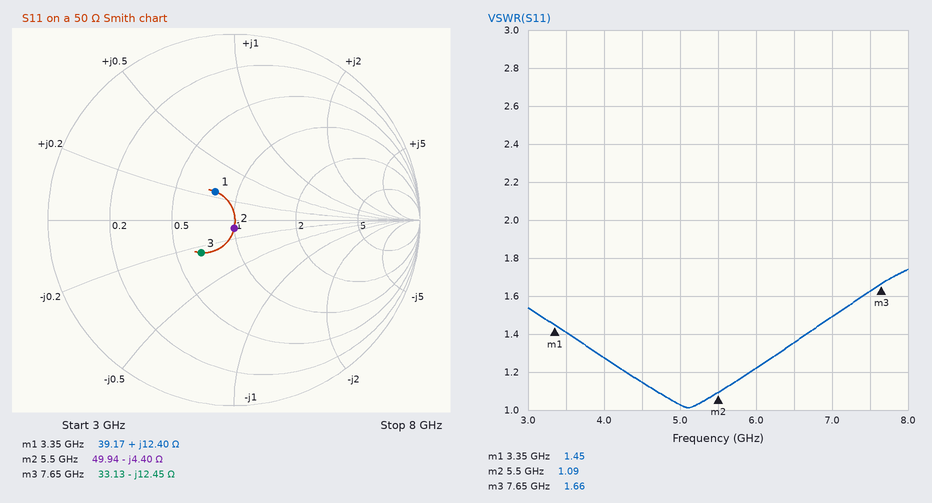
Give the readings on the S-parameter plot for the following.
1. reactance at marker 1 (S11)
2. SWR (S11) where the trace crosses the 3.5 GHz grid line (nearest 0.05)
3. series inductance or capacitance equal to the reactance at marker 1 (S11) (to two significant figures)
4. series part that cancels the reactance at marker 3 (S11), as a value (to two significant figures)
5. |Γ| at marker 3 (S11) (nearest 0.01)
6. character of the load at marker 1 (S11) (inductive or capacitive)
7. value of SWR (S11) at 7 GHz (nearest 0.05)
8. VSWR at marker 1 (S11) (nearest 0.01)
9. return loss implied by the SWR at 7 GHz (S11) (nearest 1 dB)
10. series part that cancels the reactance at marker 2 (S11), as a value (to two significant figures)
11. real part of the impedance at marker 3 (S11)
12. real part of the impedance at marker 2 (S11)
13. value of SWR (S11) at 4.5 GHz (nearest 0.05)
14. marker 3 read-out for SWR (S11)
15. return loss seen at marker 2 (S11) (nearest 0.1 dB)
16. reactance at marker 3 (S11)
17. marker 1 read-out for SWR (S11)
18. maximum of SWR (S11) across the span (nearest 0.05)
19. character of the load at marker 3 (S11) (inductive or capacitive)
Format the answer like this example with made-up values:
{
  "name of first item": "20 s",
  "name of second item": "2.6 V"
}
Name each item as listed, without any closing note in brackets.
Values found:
{
  "reactance at marker 1": "+12.40 Ω",
  "SWR (S11) where the trace crosses the 3.5 GHz grid line": "1.40",
  "series inductance or capacitance equal to the reactance at marker 1 (S11)": "590 pH",
  "series part that cancels the reactance at marker 3 (S11), as a value": "260 pH",
  "|Γ| at marker 3 (S11)": "0.25",
  "character of the load at marker 1 (S11)": "inductive",
  "value of SWR (S11) at 7 GHz": "1.50",
  "VSWR at marker 1 (S11)": "1.45",
  "return loss implied by the SWR at 7 GHz (S11)": "14 dB",
  "series part that cancels the reactance at marker 2 (S11), as a value": "130 pH",
  "real part of the impedance at marker 3": "33.13 Ω",
  "real part of the impedance at marker 2": "49.94 Ω",
  "value of SWR (S11) at 4.5 GHz": "1.15",
  "marker 3 read-out for SWR": "1.66",
  "return loss seen at marker 2 (S11)": "27.1 dB",
  "reactance at marker 3": "-12.45 Ω",
  "marker 1 read-out for SWR": "1.45",
  "maximum of SWR (S11) across the span": "1.75",
  "character of the load at marker 3 (S11)": "capacitive"
}
